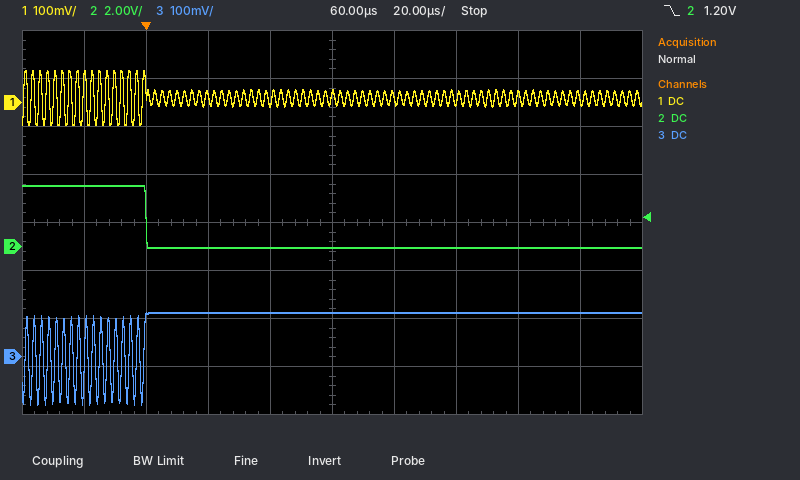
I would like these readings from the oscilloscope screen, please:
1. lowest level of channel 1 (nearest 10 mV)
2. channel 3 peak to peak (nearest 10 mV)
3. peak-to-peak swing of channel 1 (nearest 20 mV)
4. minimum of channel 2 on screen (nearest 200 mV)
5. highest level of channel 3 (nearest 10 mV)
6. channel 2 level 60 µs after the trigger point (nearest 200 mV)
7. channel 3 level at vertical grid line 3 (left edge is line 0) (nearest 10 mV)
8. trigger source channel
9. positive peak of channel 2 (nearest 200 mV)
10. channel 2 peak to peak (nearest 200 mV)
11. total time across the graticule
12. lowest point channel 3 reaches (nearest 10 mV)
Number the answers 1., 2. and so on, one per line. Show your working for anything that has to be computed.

1. -50 mV
2. 90 mV − (-100 mV) = 190 mV
3. 120 mV
4. 0.0 V
5. 90 mV
6. 0.0 V
7. 90 mV
8. channel 2
9. 2.6 V
10. 2.6 V − (0.0 V) = 2.6 V
11. 200 µs
12. -100 mV
